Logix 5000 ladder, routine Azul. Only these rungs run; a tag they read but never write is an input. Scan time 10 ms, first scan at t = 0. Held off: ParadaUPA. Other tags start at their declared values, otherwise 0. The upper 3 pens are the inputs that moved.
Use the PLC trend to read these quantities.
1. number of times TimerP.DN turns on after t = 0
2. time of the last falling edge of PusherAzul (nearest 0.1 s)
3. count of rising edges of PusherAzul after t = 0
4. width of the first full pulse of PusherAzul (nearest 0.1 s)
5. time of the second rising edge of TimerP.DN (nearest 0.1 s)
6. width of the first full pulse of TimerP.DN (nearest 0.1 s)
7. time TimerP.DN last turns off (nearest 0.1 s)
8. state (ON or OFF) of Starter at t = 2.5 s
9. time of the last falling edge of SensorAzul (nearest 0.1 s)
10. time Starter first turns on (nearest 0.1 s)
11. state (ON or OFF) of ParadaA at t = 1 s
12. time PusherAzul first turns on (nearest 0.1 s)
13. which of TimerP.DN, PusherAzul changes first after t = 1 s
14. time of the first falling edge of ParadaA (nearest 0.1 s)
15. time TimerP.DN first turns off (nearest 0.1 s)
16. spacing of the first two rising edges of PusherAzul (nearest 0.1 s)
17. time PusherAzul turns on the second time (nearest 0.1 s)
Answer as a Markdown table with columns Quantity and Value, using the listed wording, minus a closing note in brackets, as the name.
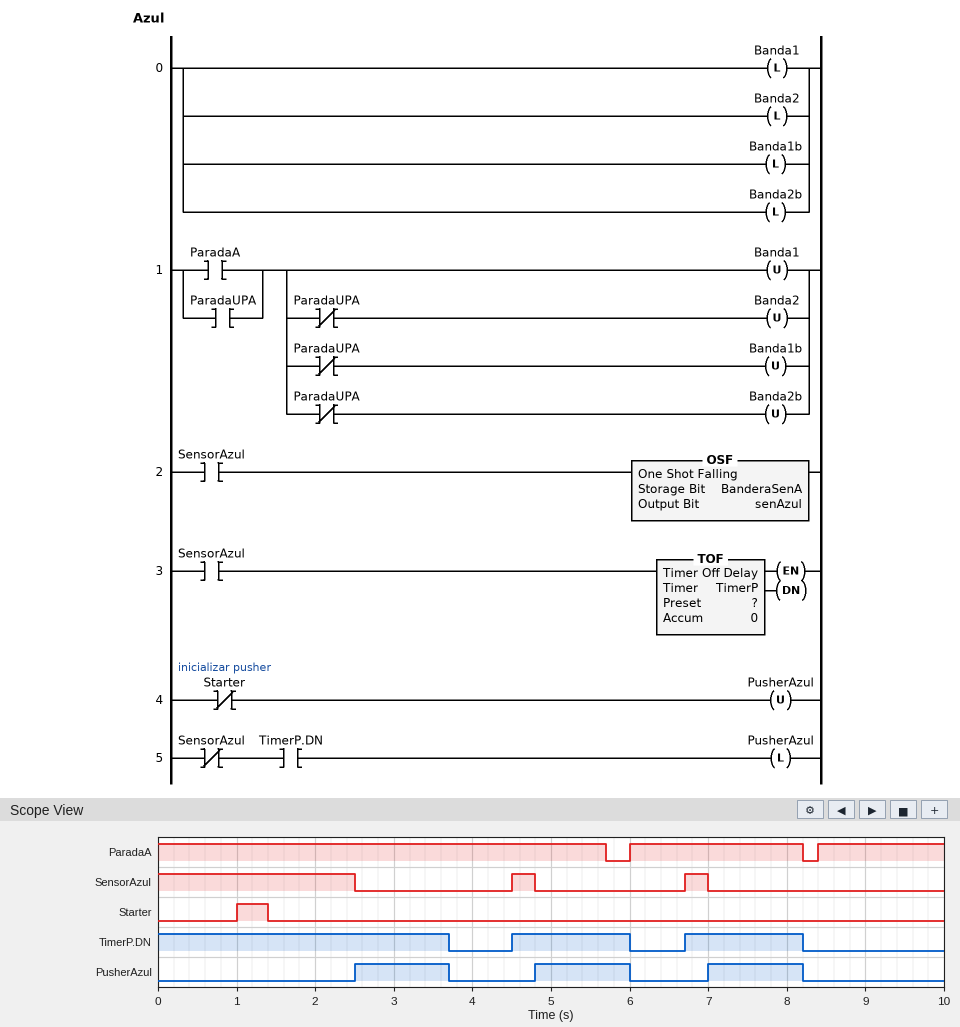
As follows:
| Quantity | Value |
|---|---|
| number of times TimerP.DN turns on after t = 0 | 2 |
| time of the last falling edge of PusherAzul | 8.2 s |
| count of rising edges of PusherAzul after t = 0 | 3 |
| width of the first full pulse of PusherAzul | 1.2 s |
| time of the second rising edge of TimerP.DN | 6.7 s |
| width of the first full pulse of TimerP.DN | 1.5 s |
| time TimerP.DN last turns off | 8.2 s |
| state (ON or OFF) of Starter at t = 2.5 s | OFF |
| time of the last falling edge of SensorAzul | 7.0 s |
| time Starter first turns on | 1.0 s |
| state (ON or OFF) of ParadaA at t = 1 s | ON |
| time PusherAzul first turns on | 2.5 s |
| which of TimerP.DN, PusherAzul changes first after t = 1 s | PusherAzul |
| time of the first falling edge of ParadaA | 5.7 s |
| time TimerP.DN first turns off | 3.7 s |
| spacing of the first two rising edges of PusherAzul | 2.3 s |
| time PusherAzul turns on the second time | 4.8 s |
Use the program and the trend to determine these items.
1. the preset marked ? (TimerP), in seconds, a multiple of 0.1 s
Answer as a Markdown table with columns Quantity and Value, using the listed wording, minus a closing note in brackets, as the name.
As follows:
| Quantity | Value |
|---|---|
| the preset marked ? (TimerP), in seconds, a multiple of 0.1 s | 1.2 s |
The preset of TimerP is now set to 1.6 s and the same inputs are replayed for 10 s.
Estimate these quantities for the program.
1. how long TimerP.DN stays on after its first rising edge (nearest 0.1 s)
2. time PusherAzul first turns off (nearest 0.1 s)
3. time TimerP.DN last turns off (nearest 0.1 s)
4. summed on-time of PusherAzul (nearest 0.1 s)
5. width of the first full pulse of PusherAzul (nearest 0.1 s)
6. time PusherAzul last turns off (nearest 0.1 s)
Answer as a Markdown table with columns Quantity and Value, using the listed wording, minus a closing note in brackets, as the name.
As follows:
| Quantity | Value |
|---|---|
| how long TimerP.DN stays on after its first rising edge | 1.9 s |
| time PusherAzul first turns off | 4.1 s |
| time TimerP.DN last turns off | 8.6 s |
| summed on-time of PusherAzul | 4.8 s |
| width of the first full pulse of PusherAzul | 1.6 s |
| time PusherAzul last turns off | 8.6 s |
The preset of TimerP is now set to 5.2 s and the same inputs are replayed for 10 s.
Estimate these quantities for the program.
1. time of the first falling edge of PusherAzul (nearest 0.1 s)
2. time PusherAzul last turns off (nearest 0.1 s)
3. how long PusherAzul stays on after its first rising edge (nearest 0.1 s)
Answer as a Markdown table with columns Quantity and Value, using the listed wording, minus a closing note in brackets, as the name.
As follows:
| Quantity | Value |
|---|---|
| time of the first falling edge of PusherAzul | 4.5 s |
| time PusherAzul last turns off | 6.7 s |
| how long PusherAzul stays on after its first rising edge | 2.0 s |
